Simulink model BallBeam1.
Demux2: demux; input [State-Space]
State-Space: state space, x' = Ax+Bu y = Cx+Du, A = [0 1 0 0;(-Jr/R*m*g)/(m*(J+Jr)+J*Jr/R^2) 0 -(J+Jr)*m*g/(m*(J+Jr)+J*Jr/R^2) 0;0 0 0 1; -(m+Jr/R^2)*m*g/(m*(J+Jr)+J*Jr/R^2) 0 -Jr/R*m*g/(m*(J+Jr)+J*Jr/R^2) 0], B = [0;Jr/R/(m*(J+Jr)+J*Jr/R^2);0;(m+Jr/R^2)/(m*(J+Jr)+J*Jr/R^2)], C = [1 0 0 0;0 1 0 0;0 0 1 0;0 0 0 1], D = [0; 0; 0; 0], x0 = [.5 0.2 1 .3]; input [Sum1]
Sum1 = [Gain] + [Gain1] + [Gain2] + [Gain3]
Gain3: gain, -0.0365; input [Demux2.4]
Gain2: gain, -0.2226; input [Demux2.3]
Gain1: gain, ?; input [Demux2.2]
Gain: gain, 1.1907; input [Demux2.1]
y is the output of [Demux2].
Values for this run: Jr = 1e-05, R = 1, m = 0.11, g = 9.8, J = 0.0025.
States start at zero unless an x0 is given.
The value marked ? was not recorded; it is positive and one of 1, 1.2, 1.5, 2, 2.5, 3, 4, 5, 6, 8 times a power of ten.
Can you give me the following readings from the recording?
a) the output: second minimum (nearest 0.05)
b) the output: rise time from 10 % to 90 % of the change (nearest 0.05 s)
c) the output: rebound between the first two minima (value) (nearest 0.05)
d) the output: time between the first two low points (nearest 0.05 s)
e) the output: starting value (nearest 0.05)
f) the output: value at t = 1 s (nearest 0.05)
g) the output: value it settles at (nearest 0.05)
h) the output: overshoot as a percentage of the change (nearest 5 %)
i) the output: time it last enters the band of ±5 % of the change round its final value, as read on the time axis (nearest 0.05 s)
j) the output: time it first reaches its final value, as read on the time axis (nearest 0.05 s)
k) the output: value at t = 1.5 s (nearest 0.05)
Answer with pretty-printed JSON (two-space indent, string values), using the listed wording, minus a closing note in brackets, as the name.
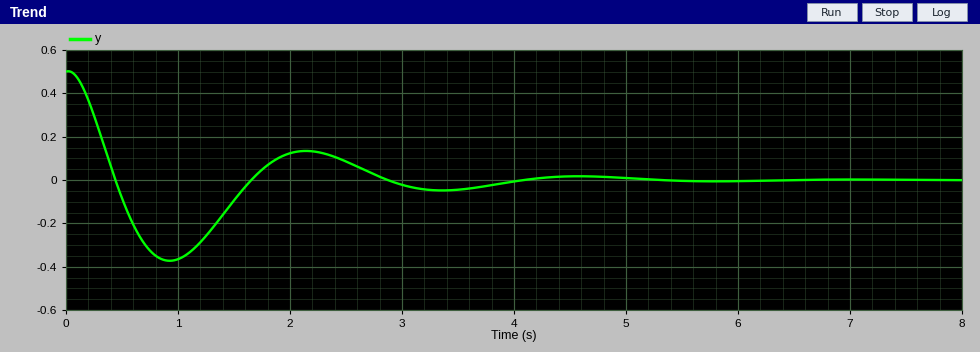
{
  "the output: second minimum": "-0.05",
  "the output: rise time from 10 % to 90 % of the change": "0.30 s",
  "the output: rebound between the first two minima (value)": "0.15",
  "the output: time between the first two low points": "2.45 s",
  "the output: starting value": "0.50",
  "the output: value at t = 1 s": "-0.35",
  "the output: value it settles at": "0.00",
  "the output: overshoot as a percentage of the change": "75 %",
  "the output: time it last enters the band of ±5 % of the change round its final value, as read on the time axis": "3.80 s",
  "the output: time it first reaches its final value, as read on the time axis": "0.45 s",
  "the output: value at t = 1.5 s": "-0.10"
}
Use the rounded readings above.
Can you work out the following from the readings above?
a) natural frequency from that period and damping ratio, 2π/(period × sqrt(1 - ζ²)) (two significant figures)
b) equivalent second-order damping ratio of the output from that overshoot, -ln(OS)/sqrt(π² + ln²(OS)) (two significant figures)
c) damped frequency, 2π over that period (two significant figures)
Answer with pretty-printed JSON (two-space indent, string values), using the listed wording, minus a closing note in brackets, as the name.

{
  "natural frequency from that period and damping ratio, 2π/(period × sqrt(1 - ζ²))": "2.6 rad/s",
  "equivalent second-order damping ratio of the output from that overshoot, -ln(OS)/sqrt(π² + ln²(OS))": "0.091",
  "damped frequency, 2π over that period": "2.6 rad/s"
}
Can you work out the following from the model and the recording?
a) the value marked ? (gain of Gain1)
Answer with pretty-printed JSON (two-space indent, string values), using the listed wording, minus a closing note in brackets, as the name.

{
  "the value marked ?": "0.05"
}
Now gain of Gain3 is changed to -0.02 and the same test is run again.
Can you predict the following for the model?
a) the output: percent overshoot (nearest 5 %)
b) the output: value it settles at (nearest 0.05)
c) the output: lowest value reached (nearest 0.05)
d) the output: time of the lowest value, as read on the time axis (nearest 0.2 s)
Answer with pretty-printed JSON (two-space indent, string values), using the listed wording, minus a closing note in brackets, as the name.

{
  "the output: percent overshoot": "20 %",
  "the output: value it settles at": "0.00",
  "the output: lowest value reached": "-0.10",
  "the output: time of the lowest value, as read on the time axis": "1.2 s"
}
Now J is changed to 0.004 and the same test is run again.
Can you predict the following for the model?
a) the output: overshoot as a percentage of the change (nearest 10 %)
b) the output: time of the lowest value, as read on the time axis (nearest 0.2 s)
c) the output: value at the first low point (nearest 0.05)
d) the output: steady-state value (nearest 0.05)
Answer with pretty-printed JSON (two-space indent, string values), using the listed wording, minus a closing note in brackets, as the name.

{
  "the output: overshoot as a percentage of the change": "80 %",
  "the output: time of the lowest value, as read on the time axis": "0.8 s",
  "the output: value at the first low point": "-0.40",
  "the output: steady-state value": "0.00"
}
